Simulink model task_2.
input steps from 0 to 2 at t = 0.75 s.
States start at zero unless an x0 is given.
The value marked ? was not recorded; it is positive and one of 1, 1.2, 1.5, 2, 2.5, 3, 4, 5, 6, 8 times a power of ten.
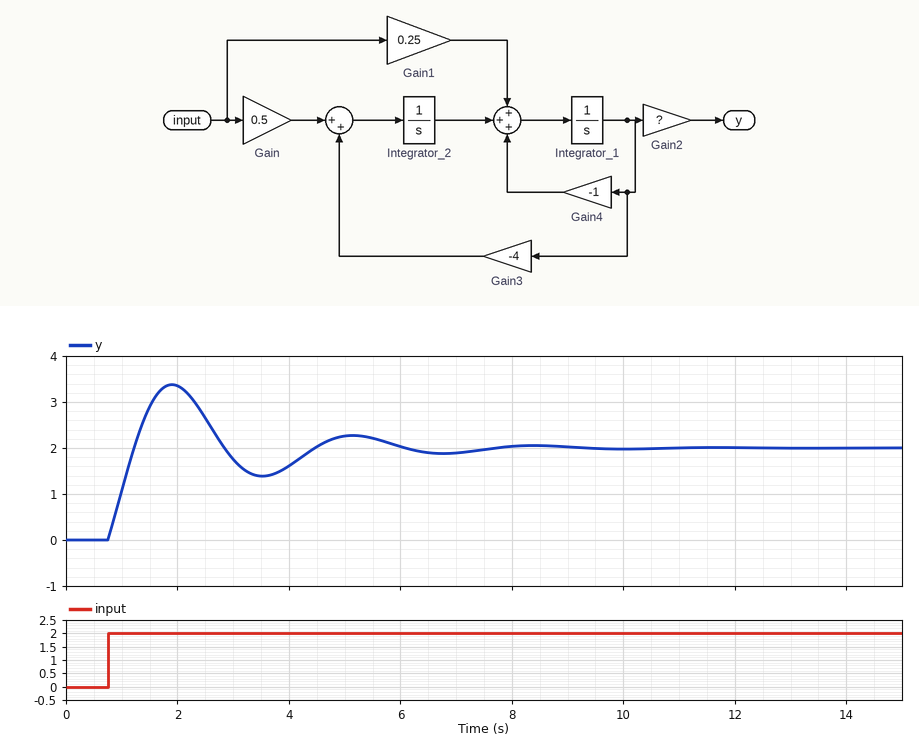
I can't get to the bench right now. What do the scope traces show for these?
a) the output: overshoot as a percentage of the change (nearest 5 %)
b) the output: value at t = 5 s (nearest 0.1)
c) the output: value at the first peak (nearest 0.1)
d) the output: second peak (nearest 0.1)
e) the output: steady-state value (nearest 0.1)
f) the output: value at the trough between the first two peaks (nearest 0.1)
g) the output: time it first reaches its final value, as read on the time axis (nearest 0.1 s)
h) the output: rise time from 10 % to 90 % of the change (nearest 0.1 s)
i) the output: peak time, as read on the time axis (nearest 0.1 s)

70 %
2.3
3.4
2.3
2.0
1.4
1.2 s
0.4 s
1.9 s
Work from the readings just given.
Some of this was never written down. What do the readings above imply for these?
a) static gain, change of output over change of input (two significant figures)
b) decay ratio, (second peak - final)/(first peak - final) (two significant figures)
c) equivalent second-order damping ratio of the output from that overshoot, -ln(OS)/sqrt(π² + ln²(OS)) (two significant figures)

1.0
0.21
0.11
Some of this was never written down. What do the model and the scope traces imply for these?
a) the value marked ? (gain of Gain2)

8
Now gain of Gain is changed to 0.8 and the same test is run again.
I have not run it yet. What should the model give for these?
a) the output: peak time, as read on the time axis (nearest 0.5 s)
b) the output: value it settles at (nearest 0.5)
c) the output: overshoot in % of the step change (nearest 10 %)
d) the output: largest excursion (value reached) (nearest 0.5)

2.0 s
3.0
50 %
5.0
